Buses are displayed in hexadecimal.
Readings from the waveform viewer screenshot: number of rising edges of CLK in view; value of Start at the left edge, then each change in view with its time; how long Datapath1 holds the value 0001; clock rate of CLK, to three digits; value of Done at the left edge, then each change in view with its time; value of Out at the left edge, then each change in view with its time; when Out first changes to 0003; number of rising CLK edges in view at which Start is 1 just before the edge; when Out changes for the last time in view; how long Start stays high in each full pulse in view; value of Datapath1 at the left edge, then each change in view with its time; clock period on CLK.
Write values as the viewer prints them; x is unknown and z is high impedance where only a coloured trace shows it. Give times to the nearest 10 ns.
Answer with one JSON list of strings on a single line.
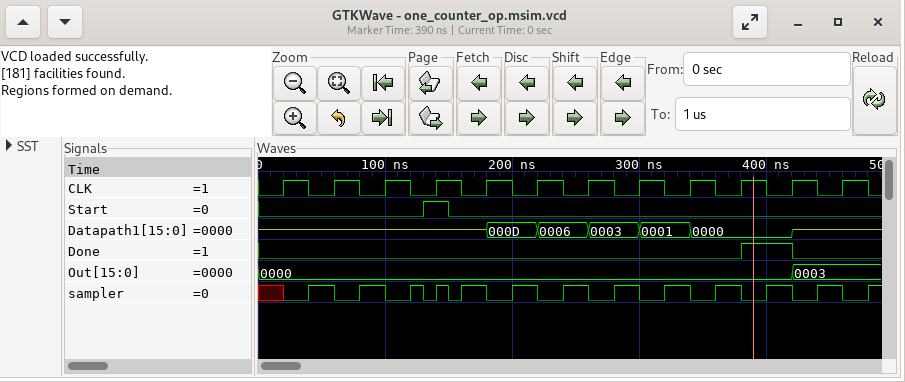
["12", "0, 1 at 130 ns, 0 at 150 ns", "40 ns", "25.0 MHz", "0, 1 at 380 ns, 0 at 420 ns", "0000, 0003 at 420 ns", "420 ns", "1", "420 ns", "20 ns", "z, 000D at 180 ns, 0006 at 220 ns, 0003 at 260 ns, 0001 at 300 ns, 0000 at 340 ns, z at 420 ns", "40 ns"]
